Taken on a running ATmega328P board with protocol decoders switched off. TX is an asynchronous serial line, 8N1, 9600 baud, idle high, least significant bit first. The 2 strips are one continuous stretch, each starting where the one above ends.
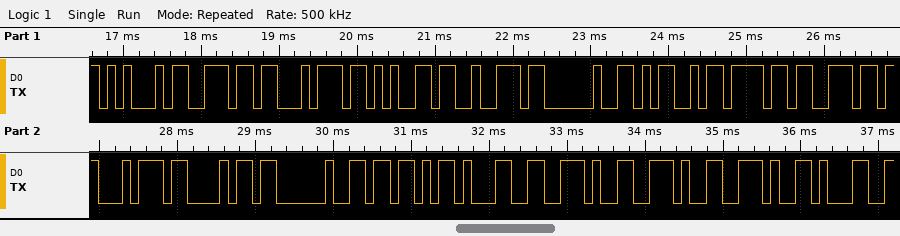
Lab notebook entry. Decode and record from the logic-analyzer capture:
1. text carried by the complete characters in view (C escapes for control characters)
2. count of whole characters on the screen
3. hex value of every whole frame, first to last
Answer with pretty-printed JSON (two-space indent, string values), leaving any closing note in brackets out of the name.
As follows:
{
  "text carried by the complete characters in view": "\"Enter Month [1...1\"",
  "count of whole characters on the screen": "18",
  "hex value of every whole frame, first to last": "0x45 0x6E 0x74 0x65 0x72 0x20 0x4D 0x6F 0x6E 0x74 0x68 0x20 0x5B 0x31 0x2E 0x2E 0x2E 0x31"
}
